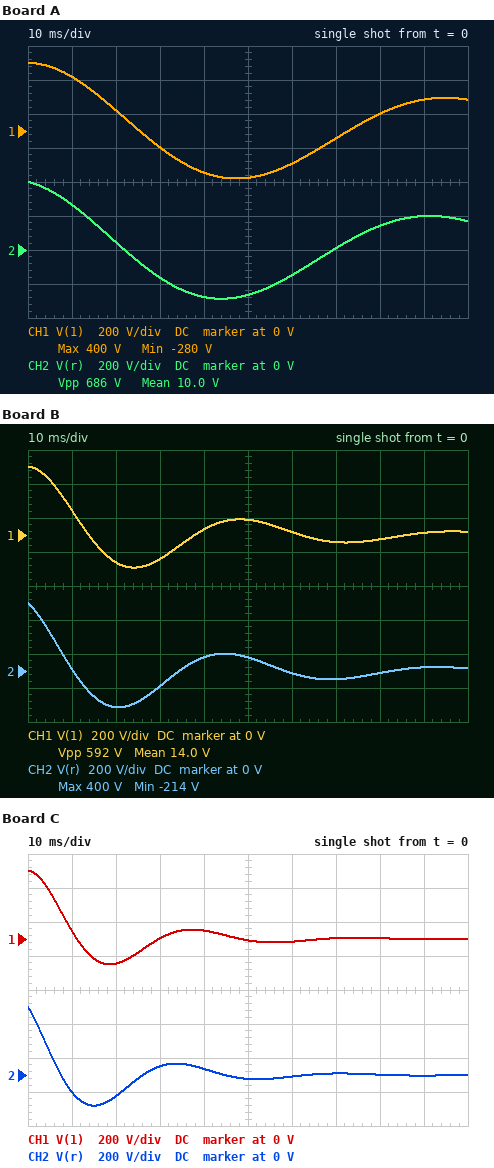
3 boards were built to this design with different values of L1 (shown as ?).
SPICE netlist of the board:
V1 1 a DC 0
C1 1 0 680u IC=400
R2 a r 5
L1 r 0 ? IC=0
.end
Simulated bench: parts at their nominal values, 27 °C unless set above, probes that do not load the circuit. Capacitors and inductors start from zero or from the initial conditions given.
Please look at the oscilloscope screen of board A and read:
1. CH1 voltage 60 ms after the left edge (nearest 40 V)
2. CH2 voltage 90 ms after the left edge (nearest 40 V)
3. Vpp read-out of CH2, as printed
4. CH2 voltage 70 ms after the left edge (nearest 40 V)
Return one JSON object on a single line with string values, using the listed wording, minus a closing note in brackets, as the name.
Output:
{"CH1 voltage 60 ms after the left edge": "-200 V", "CH2 voltage 90 ms after the left edge": "200 V", "Vpp read-out of CH2, as printed": "686 V", "CH2 voltage 70 ms after the left edge": "0 V"}
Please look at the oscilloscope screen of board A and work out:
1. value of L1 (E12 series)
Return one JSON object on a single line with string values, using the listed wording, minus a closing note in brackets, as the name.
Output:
{"value of L1": "330 mH"}
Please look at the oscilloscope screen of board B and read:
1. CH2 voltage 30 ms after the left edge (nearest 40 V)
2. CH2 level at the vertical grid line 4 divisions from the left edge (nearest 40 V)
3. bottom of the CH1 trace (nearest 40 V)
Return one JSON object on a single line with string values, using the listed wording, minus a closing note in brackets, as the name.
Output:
{"CH2 voltage 30 ms after the left edge": "-80 V", "CH2 level at the vertical grid line 4 divisions from the left edge": "80 V", "bottom of the CH1 trace": "-200 V"}
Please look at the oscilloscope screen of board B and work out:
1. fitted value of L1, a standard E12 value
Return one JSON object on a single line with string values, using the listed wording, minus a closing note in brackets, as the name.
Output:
{"fitted value of L1, a standard E12 value": "82 mH"}
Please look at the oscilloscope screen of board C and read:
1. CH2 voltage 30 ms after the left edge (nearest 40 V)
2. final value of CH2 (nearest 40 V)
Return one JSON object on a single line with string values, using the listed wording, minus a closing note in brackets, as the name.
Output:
{"CH2 voltage 30 ms after the left edge": "40 V", "final value of CH2": "0 V"}
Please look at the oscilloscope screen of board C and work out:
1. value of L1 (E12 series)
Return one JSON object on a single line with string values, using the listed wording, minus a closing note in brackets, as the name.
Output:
{"value of L1": "47 mH"}
